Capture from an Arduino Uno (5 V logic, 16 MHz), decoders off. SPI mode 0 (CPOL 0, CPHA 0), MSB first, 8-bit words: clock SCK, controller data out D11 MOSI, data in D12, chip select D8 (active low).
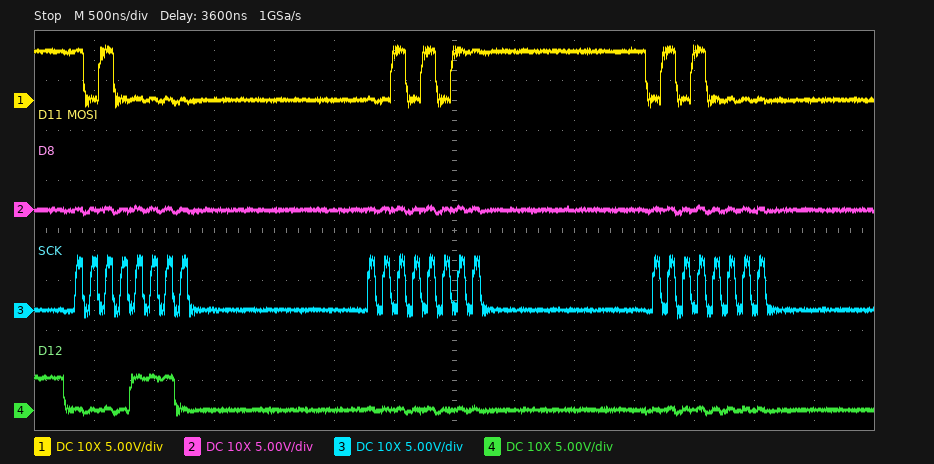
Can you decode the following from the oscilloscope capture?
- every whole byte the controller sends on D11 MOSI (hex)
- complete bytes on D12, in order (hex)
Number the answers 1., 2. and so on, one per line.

1. 0xA0 0x2B 0x50
2. 0x0E 0x00 0x00
